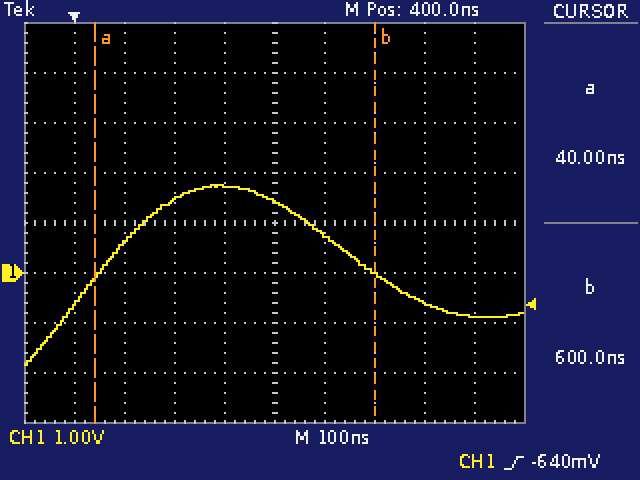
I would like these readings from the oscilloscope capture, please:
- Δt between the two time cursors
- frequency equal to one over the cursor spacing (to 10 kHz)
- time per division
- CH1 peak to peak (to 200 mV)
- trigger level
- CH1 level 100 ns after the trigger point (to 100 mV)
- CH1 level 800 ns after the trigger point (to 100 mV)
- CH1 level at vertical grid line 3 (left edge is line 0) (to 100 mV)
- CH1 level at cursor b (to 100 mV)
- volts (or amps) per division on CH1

560 ns
1.79 MHz
100 ns
3.6 V
-640 mV
600 mV
-900 mV
1.5 V
0.0 V
1 V
